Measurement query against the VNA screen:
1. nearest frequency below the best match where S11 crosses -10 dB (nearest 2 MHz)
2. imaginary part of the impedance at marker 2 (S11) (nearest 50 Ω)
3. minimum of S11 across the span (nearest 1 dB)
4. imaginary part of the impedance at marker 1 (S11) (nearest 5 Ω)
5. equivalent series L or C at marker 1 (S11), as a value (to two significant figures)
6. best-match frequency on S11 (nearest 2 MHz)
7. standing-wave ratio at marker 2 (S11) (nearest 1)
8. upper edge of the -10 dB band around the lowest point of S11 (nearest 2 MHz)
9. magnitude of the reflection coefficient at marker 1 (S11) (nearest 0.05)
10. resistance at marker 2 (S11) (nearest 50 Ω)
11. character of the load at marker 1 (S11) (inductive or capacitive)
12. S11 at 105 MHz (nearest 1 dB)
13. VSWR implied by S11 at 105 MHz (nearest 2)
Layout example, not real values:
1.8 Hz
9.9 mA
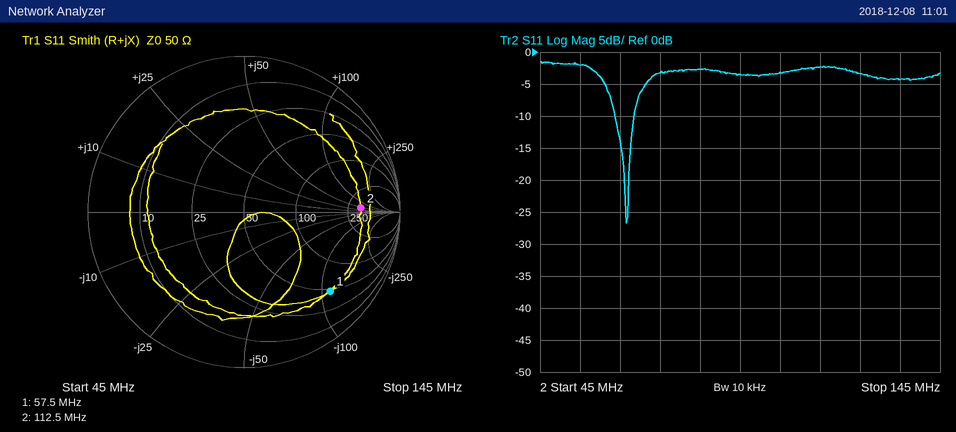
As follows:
64 MHz
+50 Ω
-27 dB
-110 Ω
25 pF
66 MHz
7
68 MHz
0.75
350 Ω
capacitive
-3 dB
6
